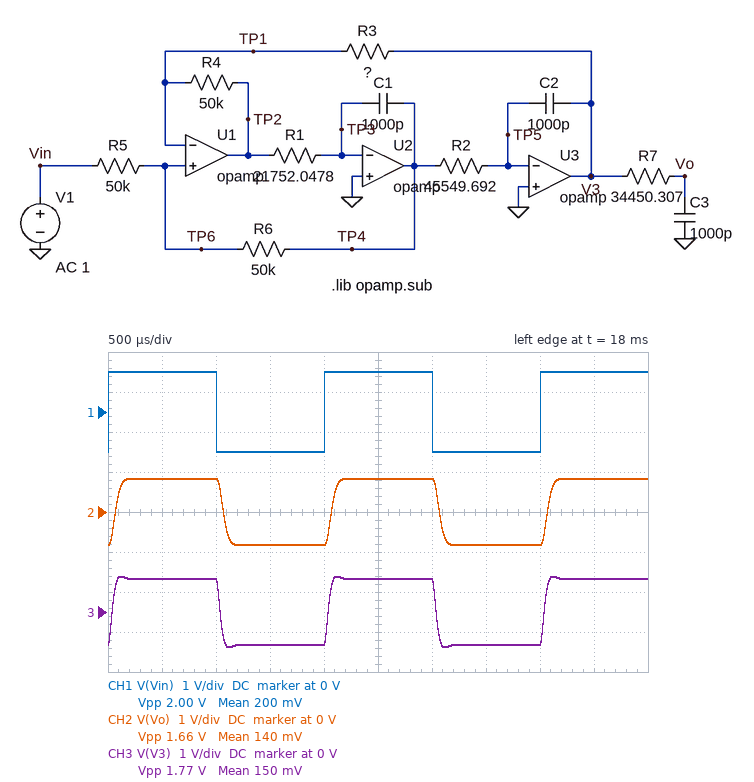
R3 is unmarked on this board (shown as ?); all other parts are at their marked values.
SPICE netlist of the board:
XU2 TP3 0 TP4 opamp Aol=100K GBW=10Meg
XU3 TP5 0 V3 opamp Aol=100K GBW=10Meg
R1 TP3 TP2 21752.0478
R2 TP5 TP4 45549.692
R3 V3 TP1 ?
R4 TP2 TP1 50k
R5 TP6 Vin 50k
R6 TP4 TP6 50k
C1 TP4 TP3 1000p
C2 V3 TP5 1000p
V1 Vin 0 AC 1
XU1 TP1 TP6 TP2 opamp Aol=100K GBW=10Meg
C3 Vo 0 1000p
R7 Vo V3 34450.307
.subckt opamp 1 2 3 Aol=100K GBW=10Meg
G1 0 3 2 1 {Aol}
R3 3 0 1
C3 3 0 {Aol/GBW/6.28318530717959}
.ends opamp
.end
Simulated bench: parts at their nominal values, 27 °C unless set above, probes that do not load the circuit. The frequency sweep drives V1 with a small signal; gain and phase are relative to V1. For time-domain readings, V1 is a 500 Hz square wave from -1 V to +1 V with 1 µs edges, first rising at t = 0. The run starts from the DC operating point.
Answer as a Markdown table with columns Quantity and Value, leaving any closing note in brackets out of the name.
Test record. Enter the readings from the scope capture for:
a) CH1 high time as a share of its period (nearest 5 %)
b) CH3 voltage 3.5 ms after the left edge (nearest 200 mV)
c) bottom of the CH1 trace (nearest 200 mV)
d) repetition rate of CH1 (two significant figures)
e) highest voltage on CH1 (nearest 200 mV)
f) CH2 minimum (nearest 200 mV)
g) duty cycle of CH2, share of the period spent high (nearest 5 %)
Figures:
| Quantity | Value |
|---|---|
| CH1 high time as a share of its period | 50 % |
| CH3 voltage 3.5 ms after the left edge | -800 mV |
| bottom of the CH1 trace | -1.0 V |
| repetition rate of CH1 | 500 Hz |
| highest voltage on CH1 | 1.0 V |
| CH2 minimum | -800 mV |
| duty cycle of CH2, share of the period spent high | 50 % |
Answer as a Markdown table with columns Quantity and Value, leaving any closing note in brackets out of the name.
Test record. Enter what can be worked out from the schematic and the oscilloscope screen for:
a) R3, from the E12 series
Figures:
| Quantity | Value |
|---|---|
| R3, from the E12 series | 33 kΩ |
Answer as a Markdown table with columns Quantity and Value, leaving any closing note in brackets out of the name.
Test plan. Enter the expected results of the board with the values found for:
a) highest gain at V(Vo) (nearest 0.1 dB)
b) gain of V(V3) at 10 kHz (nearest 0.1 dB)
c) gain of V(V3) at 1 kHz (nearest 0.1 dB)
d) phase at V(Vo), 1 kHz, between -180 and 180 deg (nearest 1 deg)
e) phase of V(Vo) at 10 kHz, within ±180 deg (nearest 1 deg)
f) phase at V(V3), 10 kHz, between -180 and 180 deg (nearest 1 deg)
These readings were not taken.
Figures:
| Quantity | Value |
|---|---|
| highest gain at V(Vo) | -1.6 dB |
| gain of V(V3) at 10 kHz | -10.7 dB |
| gain of V(V3) at 1 kHz | -1.6 dB |
| phase at V(Vo), 1 kHz, between -180 and 180 deg | -26 deg |
| phase of V(Vo) at 10 kHz, within ±180 deg | 171 deg |
| phase at V(V3), 10 kHz, between -180 and 180 deg | -124 deg |
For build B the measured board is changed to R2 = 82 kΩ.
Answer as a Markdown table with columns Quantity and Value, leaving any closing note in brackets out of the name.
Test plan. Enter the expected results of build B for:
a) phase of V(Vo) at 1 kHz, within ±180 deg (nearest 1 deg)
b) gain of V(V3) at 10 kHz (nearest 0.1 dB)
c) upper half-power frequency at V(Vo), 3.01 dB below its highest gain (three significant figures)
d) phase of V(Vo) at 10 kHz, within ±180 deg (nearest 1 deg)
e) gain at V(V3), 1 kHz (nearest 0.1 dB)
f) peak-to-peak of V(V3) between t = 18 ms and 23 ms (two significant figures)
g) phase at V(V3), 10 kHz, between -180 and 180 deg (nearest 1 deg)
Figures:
| Quantity | Value |
|---|---|
| phase of V(Vo) at 1 kHz, within ±180 deg | -36 deg |
| gain of V(V3) at 10 kHz | -16.6 dB |
| upper half-power frequency at V(Vo), 3.01 dB below its highest gain | 2.38 kHz |
| phase of V(Vo) at 10 kHz, within ±180 deg | 164 deg |
| gain at V(V3), 1 kHz | -2.0 dB |
| peak-to-peak of V(V3) between t = 18 ms and 23 ms | 1.7 V |
| phase at V(V3), 10 kHz, between -180 and 180 deg | -131 deg |
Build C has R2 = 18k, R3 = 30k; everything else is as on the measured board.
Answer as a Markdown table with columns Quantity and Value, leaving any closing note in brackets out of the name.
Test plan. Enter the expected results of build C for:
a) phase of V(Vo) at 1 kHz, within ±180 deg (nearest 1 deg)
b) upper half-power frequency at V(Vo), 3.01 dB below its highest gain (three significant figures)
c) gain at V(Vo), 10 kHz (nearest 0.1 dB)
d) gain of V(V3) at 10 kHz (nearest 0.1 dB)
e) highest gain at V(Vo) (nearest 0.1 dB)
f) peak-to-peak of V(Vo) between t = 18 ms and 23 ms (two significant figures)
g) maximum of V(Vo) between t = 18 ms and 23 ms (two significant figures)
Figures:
| Quantity | Value |
|---|---|
| phase of V(Vo) at 1 kHz, within ±180 deg | -17 deg |
| upper half-power frequency at V(Vo), 3.01 dB below its highest gain | 6.07 kHz |
| gain at V(Vo), 10 kHz | -8.6 dB |
| gain of V(V3) at 10 kHz | -1.1 dB |
| highest gain at V(Vo) | -1.9 dB |
| peak-to-peak of V(Vo) between t = 18 ms and 23 ms | 1.6 V |
| maximum of V(Vo) between t = 18 ms and 23 ms | 800 mV |
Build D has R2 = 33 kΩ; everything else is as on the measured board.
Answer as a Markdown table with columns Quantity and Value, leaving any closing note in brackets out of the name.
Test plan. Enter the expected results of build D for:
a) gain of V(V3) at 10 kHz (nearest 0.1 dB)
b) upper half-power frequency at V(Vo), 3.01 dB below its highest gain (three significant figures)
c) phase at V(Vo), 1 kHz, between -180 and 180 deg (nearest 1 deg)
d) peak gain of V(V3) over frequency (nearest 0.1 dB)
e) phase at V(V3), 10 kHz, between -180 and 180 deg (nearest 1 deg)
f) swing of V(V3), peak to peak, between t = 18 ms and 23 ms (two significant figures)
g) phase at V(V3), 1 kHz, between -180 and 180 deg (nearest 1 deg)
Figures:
| Quantity | Value |
|---|---|
| gain of V(V3) at 10 kHz | -7.3 dB |
| upper half-power frequency at V(Vo), 3.01 dB below its highest gain | 4.65 kHz |
| phase at V(Vo), 1 kHz, between -180 and 180 deg | -22 deg |
| peak gain of V(V3) over frequency | -1.4 dB |
| phase at V(V3), 10 kHz, between -180 and 180 deg | -117 deg |
| swing of V(V3), peak to peak, between t = 18 ms and 23 ms | 1.9 V |
| phase at V(V3), 1 kHz, between -180 and 180 deg | -10 deg |
